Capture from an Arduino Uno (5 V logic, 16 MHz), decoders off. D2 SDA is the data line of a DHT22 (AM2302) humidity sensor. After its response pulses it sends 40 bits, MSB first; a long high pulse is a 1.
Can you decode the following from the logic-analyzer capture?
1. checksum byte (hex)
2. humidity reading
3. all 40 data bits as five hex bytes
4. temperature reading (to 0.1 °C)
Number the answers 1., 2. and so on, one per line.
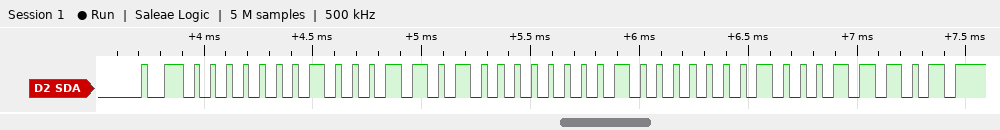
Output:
1. 0x1D
2. 28.2 %
3. 01 1A 01 01 1D
4. 25.7 °C
